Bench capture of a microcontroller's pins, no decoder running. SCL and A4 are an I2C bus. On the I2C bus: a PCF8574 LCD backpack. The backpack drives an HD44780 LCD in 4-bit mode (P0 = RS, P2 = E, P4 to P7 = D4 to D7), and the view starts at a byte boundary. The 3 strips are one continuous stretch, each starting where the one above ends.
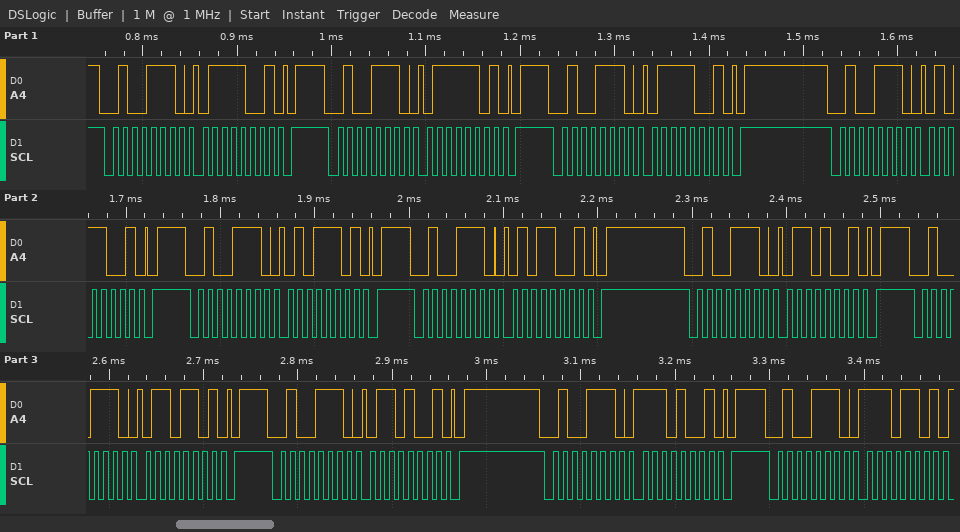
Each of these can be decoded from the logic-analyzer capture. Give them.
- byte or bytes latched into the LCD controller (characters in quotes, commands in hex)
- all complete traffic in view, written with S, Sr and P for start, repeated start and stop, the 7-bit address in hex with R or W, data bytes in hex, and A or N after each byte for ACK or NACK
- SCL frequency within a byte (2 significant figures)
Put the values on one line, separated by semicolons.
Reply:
'u'; S 27W A 79 A P S 27W A 7D A P S 27W A 79 A P S 27W A 59 A P S 27W A 5D A P S 27W A 59 A P S 27W A 69 A P S 27W A 6D A P S 27W A 69 A P S 27W A E9 A P S 27W A ED A; 100 kHz
